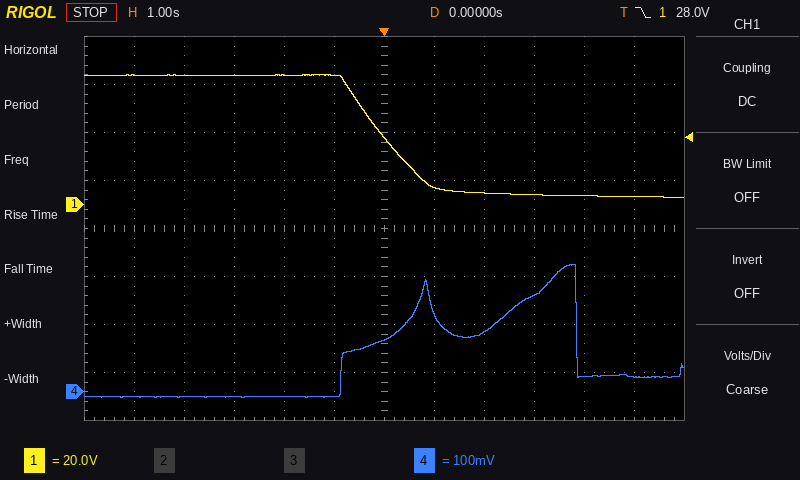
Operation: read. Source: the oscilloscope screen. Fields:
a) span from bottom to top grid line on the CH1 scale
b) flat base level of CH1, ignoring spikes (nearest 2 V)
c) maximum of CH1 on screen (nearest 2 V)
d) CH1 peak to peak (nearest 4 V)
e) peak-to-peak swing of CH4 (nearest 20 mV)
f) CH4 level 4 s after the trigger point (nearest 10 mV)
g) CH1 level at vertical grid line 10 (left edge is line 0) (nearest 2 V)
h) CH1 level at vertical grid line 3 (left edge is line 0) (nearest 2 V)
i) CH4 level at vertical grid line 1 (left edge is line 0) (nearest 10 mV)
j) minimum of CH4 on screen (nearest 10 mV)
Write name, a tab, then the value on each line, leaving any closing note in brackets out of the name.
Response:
span from bottom to top grid line on the CH1 scale	160 V
flat base level of CH1, ignoring spikes	4 V
maximum of CH1 on screen	54 V
CH1 peak to peak	52 V
peak-to-peak swing of CH4	280 mV
CH4 level 4 s after the trigger point	30 mV
CH1 level at vertical grid line 10 (left edge is line 0)	4 V
CH1 level at vertical grid line 3 (left edge is line 0)	54 V
CH4 level at vertical grid line 1 (left edge is line 0)	-10 mV
minimum of CH4 on screen	-10 mV
